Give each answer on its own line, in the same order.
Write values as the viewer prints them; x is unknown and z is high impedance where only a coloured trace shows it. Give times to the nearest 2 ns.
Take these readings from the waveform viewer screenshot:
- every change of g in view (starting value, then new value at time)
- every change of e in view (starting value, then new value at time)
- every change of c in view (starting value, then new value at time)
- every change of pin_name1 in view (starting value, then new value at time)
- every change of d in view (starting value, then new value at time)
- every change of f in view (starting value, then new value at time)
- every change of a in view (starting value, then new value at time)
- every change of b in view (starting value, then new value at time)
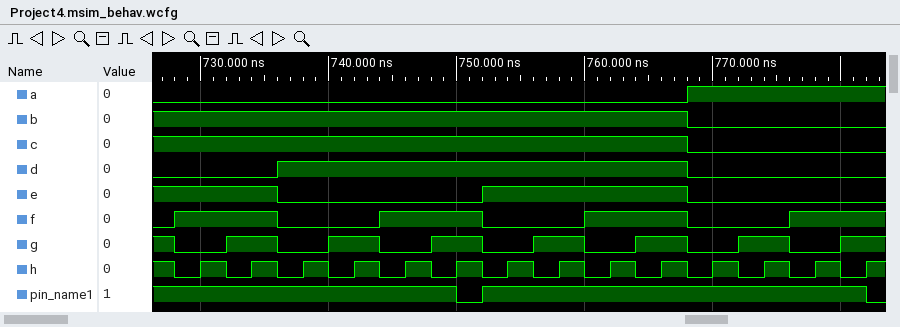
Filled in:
1, 0 at 728 ns, 1 at 732 ns, 0 at 736 ns, 1 at 740 ns, 0 at 744 ns, 1 at 748 ns, 0 at 752 ns, 1 at 756 ns, 0 at 760 ns, 1 at 764 ns, 0 at 768 ns, 1 at 772 ns, 0 at 776 ns, 1 at 780 ns
1, 0 at 736 ns, 1 at 752 ns, 0 at 768 ns
1, 0 at 768 ns
1, 0 at 750 ns, 1 at 752 ns, 0 at 782 ns
0, 1 at 736 ns, 0 at 768 ns
0, 1 at 728 ns, 0 at 736 ns, 1 at 744 ns, 0 at 752 ns, 1 at 760 ns, 0 at 768 ns, 1 at 776 ns
0, 1 at 768 ns
1, 0 at 768 ns
